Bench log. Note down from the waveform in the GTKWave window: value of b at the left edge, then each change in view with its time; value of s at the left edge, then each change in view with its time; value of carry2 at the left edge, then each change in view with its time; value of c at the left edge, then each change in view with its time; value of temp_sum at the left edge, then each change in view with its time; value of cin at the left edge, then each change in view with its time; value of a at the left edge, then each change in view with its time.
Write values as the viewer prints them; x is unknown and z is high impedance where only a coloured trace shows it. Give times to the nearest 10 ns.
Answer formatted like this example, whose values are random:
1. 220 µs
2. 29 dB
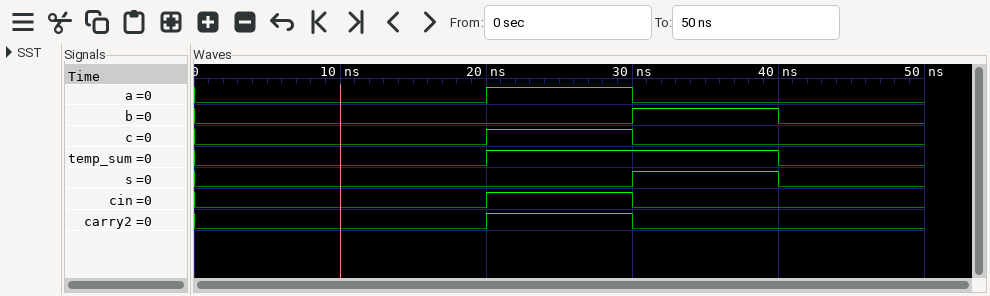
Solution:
1. 0, 1 at 30 ns, 0 at 40 ns
2. 0, 1 at 30 ns, 0 at 40 ns
3. 0, 1 at 20 ns, 0 at 30 ns
4. 0, 1 at 20 ns, 0 at 30 ns
5. 0, 1 at 20 ns, 0 at 40 ns
6. 0, 1 at 20 ns, 0 at 30 ns
7. 0, 1 at 20 ns, 0 at 30 ns
